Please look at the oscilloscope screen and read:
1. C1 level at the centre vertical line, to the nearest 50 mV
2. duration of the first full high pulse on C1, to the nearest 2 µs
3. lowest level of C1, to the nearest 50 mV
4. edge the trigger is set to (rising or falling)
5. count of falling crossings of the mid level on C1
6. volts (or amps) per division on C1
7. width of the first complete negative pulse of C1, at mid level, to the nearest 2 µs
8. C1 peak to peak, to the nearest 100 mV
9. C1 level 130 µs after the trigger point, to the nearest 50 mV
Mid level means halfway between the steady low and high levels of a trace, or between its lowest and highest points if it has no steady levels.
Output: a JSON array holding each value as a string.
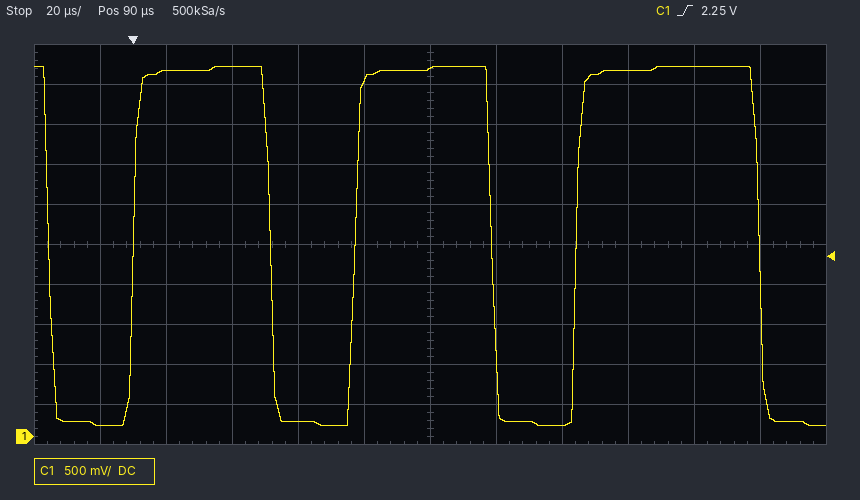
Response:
["4.60 V", "42 µs", "150 mV", "rising", "4", "500 mV", "26 µs", "4.50 V", "150 mV"]
